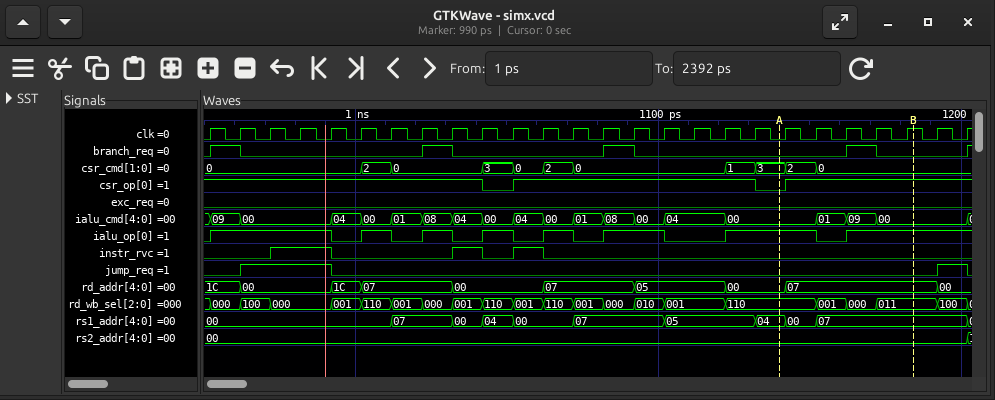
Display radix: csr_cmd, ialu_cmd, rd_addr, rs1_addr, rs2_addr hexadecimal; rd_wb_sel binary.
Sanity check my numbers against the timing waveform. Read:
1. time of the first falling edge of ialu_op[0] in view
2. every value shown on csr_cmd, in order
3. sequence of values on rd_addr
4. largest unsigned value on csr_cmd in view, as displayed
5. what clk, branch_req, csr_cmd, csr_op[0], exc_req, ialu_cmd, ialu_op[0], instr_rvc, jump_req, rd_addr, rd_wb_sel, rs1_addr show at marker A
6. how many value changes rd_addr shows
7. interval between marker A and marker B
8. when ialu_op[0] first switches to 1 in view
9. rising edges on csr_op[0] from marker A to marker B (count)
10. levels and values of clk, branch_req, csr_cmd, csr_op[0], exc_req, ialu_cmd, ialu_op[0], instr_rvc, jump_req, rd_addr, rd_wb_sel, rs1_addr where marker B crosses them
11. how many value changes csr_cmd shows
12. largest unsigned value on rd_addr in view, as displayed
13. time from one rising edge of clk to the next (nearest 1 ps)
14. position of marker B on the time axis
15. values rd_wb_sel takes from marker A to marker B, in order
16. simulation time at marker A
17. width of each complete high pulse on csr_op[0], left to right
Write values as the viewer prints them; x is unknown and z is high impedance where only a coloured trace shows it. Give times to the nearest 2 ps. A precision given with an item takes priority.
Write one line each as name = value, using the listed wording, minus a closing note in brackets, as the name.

time of the first falling edge of ialu_op[0] in view = 992 ps
every value shown on csr_cmd, in order = 0, 2, 0, 3, 0, 2, 0, 1, 3, 2, 0
sequence of values on rd_addr = 1C, 00, 1C, 07, 00, 07, 05, 00, 07, 00
largest unsigned value on csr_cmd in view, as displayed = 3
what clk, branch_req, csr_cmd, csr_op[0], exc_req, ialu_cmd, ialu_op[0], instr_rvc, jump_req, rd_addr, rd_wb_sel, rs1_addr show at marker A = clk=0, branch_req=0, csr_cmd=3, csr_op[0]=0, exc_req=0, ialu_cmd=00, ialu_op[0]=1, instr_rvc=0, jump_req=0, rd_addr=00, rd_wb_sel=110, rs1_addr=04
how many value changes rd_addr shows = 9
interval between marker A and marker B = 44 ps
when ialu_op[0] first switches to 1 in view = 952 ps
rising edges on csr_op[0] from marker A to marker B = 1
levels and values of clk, branch_req, csr_cmd, csr_op[0], exc_req, ialu_cmd, ialu_op[0], instr_rvc, jump_req, rd_addr, rd_wb_sel, rs1_addr where marker B crosses them = clk=1, branch_req=0, csr_cmd=0, csr_op[0]=1, exc_req=0, ialu_cmd=00, ialu_op[0]=1, instr_rvc=0, jump_req=0, rd_addr=07, rd_wb_sel=011, rs1_addr=07
how many value changes csr_cmd shows = 10
largest unsigned value on rd_addr in view, as displayed = 1C
time from one rising edge of clk to the next = 10 ps
position of marker B on the time axis = 1184 ps
values rd_wb_sel takes from marker A to marker B, in order = 110, 001, 000, 011
simulation time at marker A = 1140 ps
width of each complete high pulse on csr_op[0], left to right = 80 ps
